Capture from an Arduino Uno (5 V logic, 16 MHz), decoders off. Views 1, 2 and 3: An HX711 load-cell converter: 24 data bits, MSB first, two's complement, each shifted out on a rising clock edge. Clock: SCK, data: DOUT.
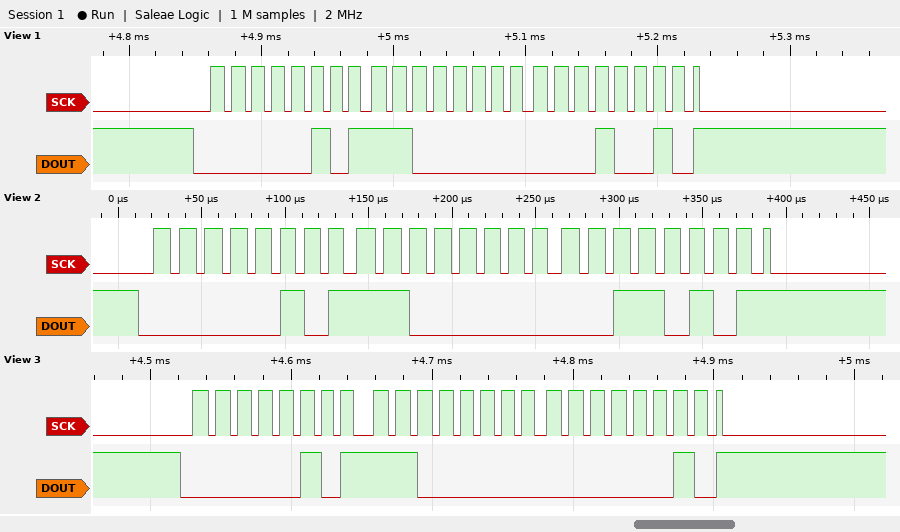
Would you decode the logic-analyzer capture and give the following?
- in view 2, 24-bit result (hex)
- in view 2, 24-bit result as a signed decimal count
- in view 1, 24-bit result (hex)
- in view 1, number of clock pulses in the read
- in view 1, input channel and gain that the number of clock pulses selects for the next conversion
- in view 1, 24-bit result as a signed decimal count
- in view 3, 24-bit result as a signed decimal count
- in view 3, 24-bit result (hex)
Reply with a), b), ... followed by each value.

a) 0x05C035
b) 376885
c) 0x05C012
d) 25
e) channel A, gain 128
f) 376850
g) 376834
h) 0x05C002
